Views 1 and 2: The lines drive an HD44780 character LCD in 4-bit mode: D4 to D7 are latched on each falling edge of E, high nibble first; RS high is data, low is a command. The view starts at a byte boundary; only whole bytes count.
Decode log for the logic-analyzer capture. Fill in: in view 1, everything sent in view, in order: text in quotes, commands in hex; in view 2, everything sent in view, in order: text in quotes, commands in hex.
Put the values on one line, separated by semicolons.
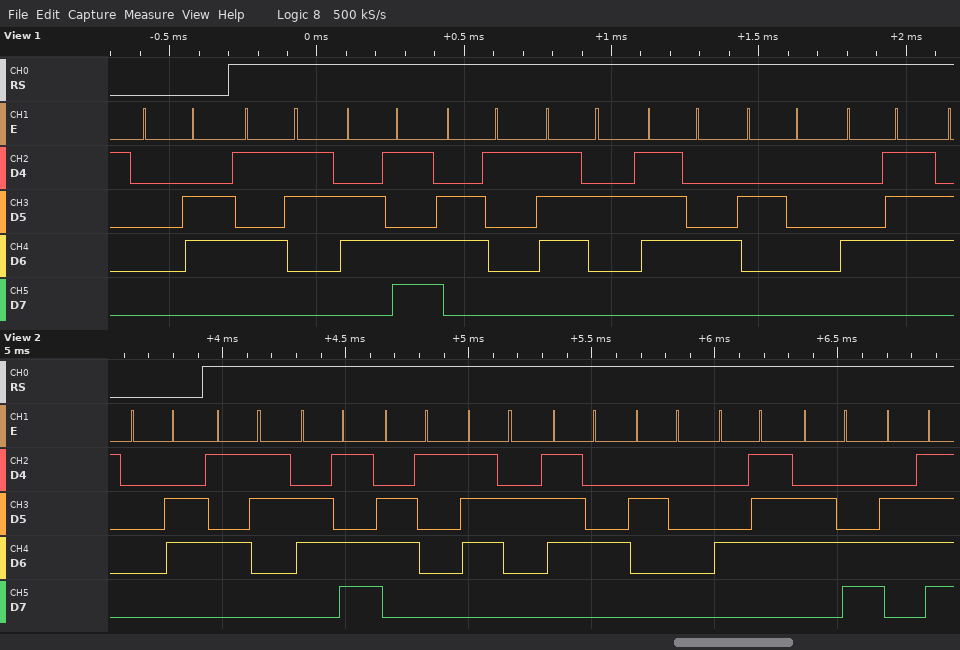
0x06 "Smart G"; 0x06 "Smart Glo"
